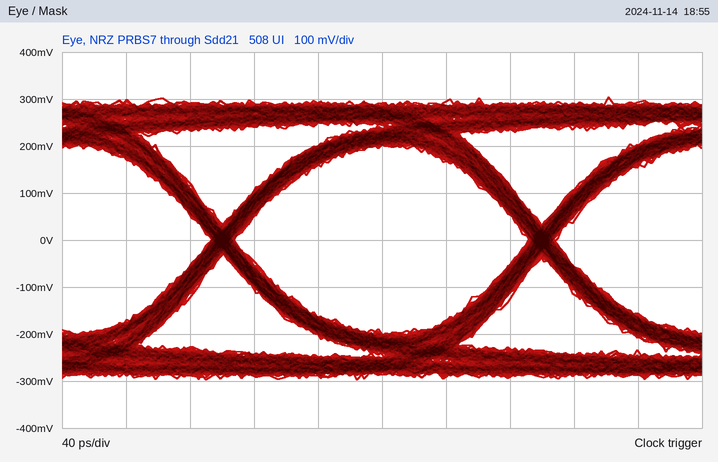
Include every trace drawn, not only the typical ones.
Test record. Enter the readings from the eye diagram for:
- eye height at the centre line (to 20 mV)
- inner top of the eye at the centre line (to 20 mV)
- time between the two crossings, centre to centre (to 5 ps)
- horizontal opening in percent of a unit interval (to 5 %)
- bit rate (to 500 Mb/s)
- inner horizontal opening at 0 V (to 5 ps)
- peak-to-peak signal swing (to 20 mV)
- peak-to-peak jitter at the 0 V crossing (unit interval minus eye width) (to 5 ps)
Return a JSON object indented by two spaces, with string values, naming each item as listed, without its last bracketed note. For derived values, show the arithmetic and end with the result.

{
  "eye height at the centre line": "400 mV",
  "inner top of the eye at the centre line": "200 mV",
  "time between the two crossings, centre to centre": "200 ps",
  "horizontal opening in percent of a unit interval": "185 ps / 200 ps ≈ 92.5 %, so 90 % to the nearest 5 %",
  "bit rate": "5.0 Gb/s",
  "inner horizontal opening at 0 V": "185 ps",
  "peak-to-peak signal swing": "600 mV",
  "peak-to-peak jitter at the 0 V crossing (unit interval minus eye width)": "15 ps"
}
